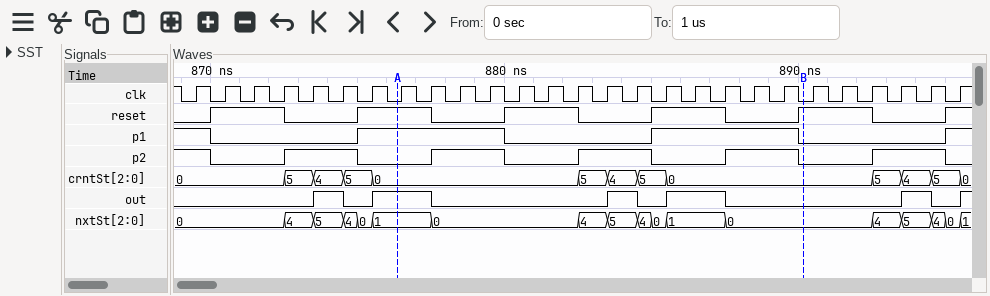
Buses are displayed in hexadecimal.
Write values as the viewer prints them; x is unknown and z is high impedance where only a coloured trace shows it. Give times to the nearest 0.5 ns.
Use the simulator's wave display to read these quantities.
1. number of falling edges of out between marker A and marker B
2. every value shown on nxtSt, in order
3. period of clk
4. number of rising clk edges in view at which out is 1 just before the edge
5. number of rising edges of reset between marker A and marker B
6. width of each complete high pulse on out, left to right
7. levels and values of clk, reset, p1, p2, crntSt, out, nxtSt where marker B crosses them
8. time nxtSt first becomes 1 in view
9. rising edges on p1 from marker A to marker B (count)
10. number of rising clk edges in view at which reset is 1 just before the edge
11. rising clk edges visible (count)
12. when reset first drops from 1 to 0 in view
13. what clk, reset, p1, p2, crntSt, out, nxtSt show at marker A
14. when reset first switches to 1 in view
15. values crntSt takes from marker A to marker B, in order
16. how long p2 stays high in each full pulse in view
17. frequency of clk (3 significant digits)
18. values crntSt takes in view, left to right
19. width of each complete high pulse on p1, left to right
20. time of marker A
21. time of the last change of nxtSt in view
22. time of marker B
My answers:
3
0, 4, 5, 4, 0, 1, 0, 4, 5, 4, 0, 1, 0, 4, 5, 4, 0, 1
1 ns
7
3
1 ns, 2 ns, 1 ns, 2 ns, 1 ns
clk=0, reset=1, p1=0, p2=0, crntSt=0, out=0, nxtSt=0
875.5 ns
1
16
27
872.5 ns
clk=0, reset=1, p1=1, p2=0, crntSt=0, out=1, nxtSt=1
870 ns
0, 5, 4, 5, 0
2.5 ns, 2.5 ns, 2.5 ns, 2.5 ns, 2.5 ns
1.00 GHz
0, 5, 4, 5, 0, 5, 4, 5, 0, 5, 4, 5, 0
5 ns, 5 ns
876.5 ns
895.5 ns
890 ns
